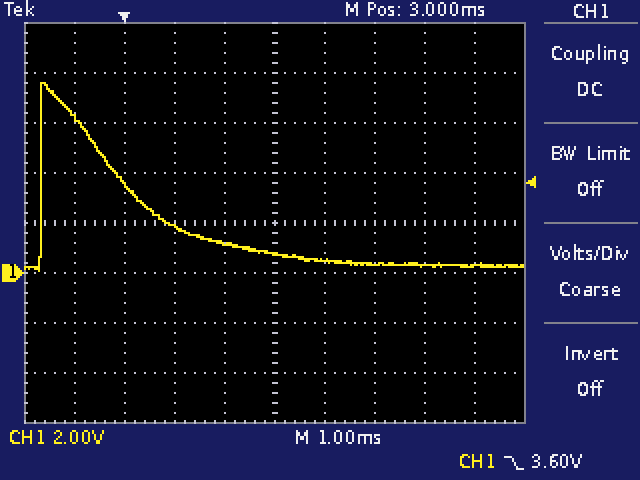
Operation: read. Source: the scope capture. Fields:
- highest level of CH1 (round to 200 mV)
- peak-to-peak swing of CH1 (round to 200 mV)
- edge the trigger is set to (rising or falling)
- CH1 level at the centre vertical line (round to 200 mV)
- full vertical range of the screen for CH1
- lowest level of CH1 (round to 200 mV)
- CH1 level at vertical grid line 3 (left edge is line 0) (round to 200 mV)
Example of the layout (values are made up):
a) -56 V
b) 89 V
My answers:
a) 7.6 V
b) 7.6 V
c) falling
d) 800 mV
e) 16 V
f) 0.0 V
g) 1.8 V
